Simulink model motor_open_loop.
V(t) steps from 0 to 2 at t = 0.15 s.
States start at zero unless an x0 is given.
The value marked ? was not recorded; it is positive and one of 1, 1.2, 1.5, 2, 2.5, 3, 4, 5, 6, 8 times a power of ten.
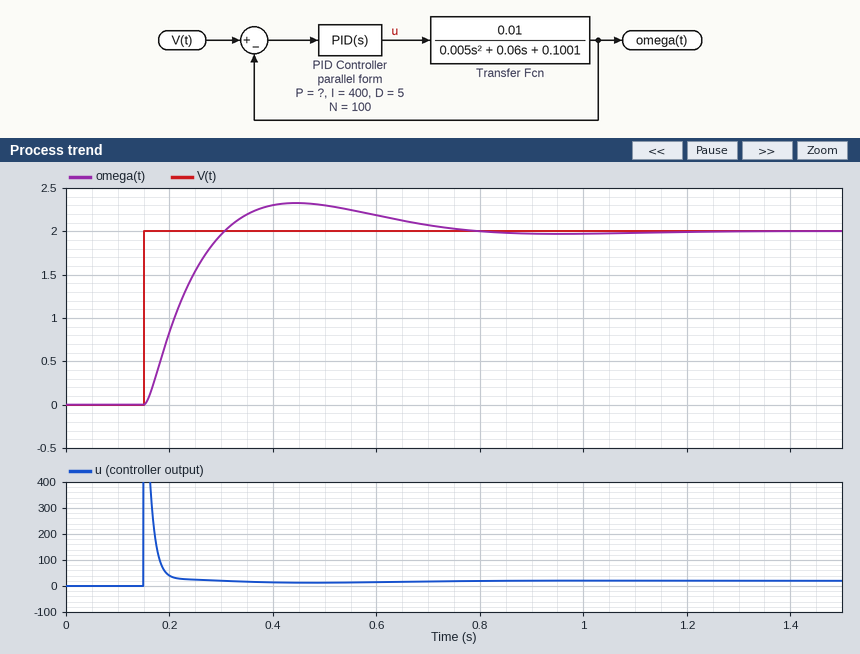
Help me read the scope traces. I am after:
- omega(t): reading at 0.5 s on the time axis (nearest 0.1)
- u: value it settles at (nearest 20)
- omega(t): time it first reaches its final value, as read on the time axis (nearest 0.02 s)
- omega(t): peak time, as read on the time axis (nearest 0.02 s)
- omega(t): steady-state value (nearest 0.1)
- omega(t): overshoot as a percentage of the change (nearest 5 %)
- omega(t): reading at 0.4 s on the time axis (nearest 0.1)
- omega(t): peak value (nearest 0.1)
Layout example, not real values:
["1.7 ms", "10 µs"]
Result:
["2.3", "20", "0.30 s", "0.44 s", "2.0", "15 %", "2.3", "2.3"]
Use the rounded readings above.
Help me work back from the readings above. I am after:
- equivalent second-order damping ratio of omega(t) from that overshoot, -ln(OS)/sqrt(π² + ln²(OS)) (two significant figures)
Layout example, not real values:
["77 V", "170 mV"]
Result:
["0.52"]
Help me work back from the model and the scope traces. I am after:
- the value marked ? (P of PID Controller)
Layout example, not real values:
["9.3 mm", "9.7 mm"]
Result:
["80"]
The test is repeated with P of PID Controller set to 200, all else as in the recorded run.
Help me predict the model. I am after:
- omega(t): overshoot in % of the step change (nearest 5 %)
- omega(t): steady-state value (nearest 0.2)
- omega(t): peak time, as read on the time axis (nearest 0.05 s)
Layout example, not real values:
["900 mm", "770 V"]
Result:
["20 %", "2.0", "0.30 s"]
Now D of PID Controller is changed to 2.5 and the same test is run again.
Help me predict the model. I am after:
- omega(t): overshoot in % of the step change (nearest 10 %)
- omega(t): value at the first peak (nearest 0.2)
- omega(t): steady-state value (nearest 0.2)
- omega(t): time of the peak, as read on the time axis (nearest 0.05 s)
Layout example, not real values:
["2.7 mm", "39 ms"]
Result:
["30 %", "2.6", "2.0", "0.40 s"]
